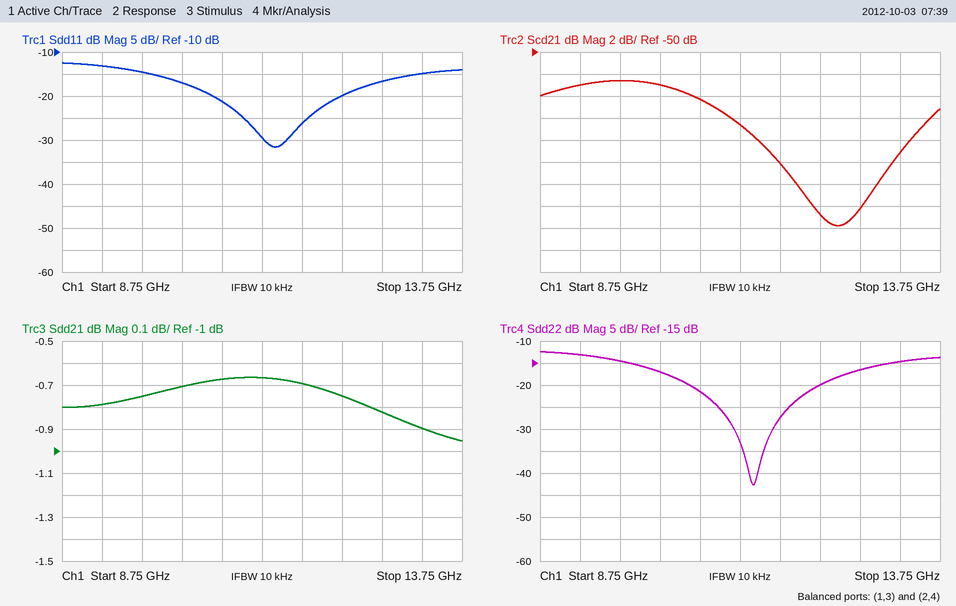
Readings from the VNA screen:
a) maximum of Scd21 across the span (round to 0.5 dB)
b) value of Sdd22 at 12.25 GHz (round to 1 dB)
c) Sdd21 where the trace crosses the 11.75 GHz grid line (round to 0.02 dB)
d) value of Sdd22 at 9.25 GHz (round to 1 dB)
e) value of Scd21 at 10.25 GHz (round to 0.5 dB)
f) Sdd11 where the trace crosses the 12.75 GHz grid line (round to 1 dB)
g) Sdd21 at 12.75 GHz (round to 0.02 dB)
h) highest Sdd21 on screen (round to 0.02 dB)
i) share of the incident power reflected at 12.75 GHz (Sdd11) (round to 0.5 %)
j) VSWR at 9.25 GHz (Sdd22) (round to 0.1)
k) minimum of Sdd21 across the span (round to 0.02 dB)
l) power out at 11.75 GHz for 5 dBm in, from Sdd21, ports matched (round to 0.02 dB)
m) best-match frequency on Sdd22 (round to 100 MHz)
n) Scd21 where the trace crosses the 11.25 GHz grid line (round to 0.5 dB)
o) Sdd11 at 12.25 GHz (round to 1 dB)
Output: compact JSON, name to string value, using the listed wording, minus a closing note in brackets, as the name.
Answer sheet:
{"maximum of Scd21 across the span": "-52.5 dB", "value of Sdd22 at 12.25 GHz": "-20 dB", "Sdd21 where the trace crosses the 11.75 GHz grid line": "-0.70 dB", "value of Sdd22 at 9.25 GHz": "-13 dB", "value of Scd21 at 10.25 GHz": "-53.0 dB", "Sdd11 where the trace crosses the 12.75 GHz grid line": "-17 dB", "Sdd21 at 12.75 GHz": "-0.82 dB", "highest Sdd21 on screen": "-0.66 dB", "share of the incident power reflected at 12.75 GHz (Sdd11)": "2.0 %", "VSWR at 9.25 GHz (Sdd22)": "1.6", "minimum of Sdd21 across the span": "-0.96 dB", "power out at 11.75 GHz for 5 dBm in, from Sdd21, ports matched": "4.30 dBm", "best-match frequency on Sdd22": "11.4 GHz", "Scd21 where the trace crosses the 11.25 GHz grid line": "-56.5 dB", "Sdd11 at 12.25 GHz": "-20 dB"}
